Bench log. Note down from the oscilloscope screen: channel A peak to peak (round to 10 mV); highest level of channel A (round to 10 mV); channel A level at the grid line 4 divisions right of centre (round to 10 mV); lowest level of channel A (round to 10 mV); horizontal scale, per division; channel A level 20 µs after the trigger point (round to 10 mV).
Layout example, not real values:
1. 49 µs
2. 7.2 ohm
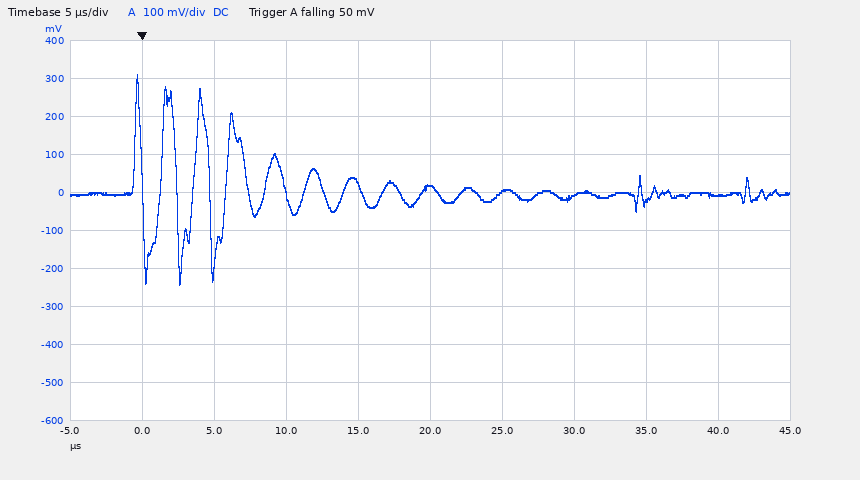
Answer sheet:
1. 550 mV
2. 310 mV
3. -10 mV
4. -240 mV
5. 5 µs
6. 20 mV
